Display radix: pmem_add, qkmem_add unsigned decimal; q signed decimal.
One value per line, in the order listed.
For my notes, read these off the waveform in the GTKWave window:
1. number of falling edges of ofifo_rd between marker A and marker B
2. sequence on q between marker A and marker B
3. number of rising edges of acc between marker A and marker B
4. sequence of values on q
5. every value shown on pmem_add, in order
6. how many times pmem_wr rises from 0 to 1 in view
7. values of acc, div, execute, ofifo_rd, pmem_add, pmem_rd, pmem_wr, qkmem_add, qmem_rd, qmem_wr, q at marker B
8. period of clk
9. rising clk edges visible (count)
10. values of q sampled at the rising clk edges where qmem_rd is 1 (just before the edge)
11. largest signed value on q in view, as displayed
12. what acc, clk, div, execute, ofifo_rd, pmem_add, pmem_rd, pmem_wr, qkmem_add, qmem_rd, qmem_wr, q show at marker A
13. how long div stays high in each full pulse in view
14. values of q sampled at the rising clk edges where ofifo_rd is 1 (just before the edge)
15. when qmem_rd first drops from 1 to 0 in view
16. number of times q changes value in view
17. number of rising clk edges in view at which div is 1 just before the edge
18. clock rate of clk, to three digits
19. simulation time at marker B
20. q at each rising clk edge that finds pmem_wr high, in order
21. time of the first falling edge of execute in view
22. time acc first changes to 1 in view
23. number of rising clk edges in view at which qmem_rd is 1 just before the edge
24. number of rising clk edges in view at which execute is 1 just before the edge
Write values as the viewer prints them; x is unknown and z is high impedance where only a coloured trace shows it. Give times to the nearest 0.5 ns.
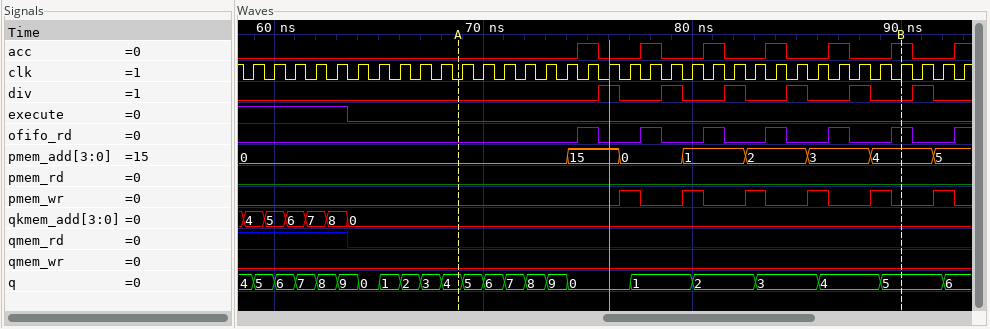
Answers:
5
4, 5, 6, 7, 8, 9, 0, 1, 2, 3, 4, 5
6
4, 5, 6, 7, 8, 9, 0, 1, 2, 3, 4, 5, 6, 7, 8, 9, 0, 1, 2, 3, 4, 5, 6
0, 15, 0, 1, 2, 3, 4, 5
6
acc=1, div=0, execute=0, ofifo_rd=1, pmem_add=4, pmem_rd=0, pmem_wr=0, qkmem_add=0, qmem_rd=0, qmem_wr=0, q=5
1 ns
35
4, 5, 6, 7, 8
9
acc=0, clk=0, div=0, execute=0, ofifo_rd=0, pmem_add=0, pmem_rd=0, pmem_wr=0, qkmem_add=0, qmem_rd=0, qmem_wr=0, q=4
1 ns, 1 ns, 1 ns, 1 ns, 1 ns, 1 ns
0, 1, 2, 3, 4, 5, 6
63.5 ns
22
6
1.00 GHz
90 ns
0, 1, 2, 3, 4, 5
63.5 ns
74.5 ns
5
5
